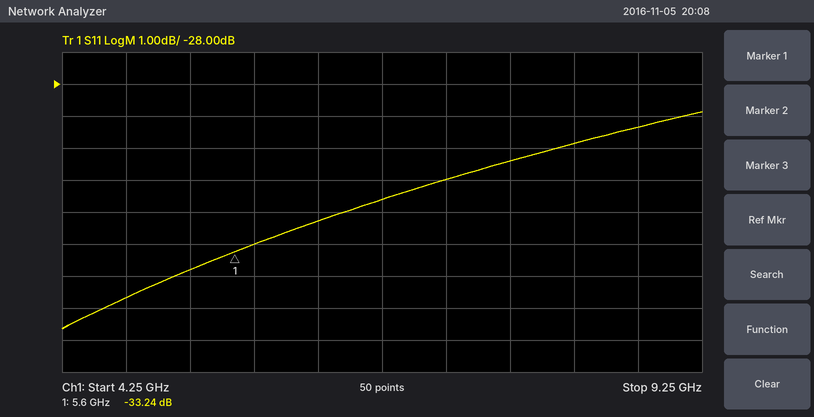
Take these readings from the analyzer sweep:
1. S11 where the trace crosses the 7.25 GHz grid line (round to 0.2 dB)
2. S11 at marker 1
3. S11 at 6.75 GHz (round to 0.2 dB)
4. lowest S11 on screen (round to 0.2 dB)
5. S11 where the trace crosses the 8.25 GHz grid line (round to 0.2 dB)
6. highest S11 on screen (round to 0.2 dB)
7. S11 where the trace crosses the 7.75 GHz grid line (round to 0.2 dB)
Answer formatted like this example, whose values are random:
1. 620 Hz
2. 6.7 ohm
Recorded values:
1. -31.0 dB
2. -33.24 dB
3. -31.6 dB
4. -35.6 dB
5. -29.8 dB
6. -28.8 dB
7. -30.4 dB
